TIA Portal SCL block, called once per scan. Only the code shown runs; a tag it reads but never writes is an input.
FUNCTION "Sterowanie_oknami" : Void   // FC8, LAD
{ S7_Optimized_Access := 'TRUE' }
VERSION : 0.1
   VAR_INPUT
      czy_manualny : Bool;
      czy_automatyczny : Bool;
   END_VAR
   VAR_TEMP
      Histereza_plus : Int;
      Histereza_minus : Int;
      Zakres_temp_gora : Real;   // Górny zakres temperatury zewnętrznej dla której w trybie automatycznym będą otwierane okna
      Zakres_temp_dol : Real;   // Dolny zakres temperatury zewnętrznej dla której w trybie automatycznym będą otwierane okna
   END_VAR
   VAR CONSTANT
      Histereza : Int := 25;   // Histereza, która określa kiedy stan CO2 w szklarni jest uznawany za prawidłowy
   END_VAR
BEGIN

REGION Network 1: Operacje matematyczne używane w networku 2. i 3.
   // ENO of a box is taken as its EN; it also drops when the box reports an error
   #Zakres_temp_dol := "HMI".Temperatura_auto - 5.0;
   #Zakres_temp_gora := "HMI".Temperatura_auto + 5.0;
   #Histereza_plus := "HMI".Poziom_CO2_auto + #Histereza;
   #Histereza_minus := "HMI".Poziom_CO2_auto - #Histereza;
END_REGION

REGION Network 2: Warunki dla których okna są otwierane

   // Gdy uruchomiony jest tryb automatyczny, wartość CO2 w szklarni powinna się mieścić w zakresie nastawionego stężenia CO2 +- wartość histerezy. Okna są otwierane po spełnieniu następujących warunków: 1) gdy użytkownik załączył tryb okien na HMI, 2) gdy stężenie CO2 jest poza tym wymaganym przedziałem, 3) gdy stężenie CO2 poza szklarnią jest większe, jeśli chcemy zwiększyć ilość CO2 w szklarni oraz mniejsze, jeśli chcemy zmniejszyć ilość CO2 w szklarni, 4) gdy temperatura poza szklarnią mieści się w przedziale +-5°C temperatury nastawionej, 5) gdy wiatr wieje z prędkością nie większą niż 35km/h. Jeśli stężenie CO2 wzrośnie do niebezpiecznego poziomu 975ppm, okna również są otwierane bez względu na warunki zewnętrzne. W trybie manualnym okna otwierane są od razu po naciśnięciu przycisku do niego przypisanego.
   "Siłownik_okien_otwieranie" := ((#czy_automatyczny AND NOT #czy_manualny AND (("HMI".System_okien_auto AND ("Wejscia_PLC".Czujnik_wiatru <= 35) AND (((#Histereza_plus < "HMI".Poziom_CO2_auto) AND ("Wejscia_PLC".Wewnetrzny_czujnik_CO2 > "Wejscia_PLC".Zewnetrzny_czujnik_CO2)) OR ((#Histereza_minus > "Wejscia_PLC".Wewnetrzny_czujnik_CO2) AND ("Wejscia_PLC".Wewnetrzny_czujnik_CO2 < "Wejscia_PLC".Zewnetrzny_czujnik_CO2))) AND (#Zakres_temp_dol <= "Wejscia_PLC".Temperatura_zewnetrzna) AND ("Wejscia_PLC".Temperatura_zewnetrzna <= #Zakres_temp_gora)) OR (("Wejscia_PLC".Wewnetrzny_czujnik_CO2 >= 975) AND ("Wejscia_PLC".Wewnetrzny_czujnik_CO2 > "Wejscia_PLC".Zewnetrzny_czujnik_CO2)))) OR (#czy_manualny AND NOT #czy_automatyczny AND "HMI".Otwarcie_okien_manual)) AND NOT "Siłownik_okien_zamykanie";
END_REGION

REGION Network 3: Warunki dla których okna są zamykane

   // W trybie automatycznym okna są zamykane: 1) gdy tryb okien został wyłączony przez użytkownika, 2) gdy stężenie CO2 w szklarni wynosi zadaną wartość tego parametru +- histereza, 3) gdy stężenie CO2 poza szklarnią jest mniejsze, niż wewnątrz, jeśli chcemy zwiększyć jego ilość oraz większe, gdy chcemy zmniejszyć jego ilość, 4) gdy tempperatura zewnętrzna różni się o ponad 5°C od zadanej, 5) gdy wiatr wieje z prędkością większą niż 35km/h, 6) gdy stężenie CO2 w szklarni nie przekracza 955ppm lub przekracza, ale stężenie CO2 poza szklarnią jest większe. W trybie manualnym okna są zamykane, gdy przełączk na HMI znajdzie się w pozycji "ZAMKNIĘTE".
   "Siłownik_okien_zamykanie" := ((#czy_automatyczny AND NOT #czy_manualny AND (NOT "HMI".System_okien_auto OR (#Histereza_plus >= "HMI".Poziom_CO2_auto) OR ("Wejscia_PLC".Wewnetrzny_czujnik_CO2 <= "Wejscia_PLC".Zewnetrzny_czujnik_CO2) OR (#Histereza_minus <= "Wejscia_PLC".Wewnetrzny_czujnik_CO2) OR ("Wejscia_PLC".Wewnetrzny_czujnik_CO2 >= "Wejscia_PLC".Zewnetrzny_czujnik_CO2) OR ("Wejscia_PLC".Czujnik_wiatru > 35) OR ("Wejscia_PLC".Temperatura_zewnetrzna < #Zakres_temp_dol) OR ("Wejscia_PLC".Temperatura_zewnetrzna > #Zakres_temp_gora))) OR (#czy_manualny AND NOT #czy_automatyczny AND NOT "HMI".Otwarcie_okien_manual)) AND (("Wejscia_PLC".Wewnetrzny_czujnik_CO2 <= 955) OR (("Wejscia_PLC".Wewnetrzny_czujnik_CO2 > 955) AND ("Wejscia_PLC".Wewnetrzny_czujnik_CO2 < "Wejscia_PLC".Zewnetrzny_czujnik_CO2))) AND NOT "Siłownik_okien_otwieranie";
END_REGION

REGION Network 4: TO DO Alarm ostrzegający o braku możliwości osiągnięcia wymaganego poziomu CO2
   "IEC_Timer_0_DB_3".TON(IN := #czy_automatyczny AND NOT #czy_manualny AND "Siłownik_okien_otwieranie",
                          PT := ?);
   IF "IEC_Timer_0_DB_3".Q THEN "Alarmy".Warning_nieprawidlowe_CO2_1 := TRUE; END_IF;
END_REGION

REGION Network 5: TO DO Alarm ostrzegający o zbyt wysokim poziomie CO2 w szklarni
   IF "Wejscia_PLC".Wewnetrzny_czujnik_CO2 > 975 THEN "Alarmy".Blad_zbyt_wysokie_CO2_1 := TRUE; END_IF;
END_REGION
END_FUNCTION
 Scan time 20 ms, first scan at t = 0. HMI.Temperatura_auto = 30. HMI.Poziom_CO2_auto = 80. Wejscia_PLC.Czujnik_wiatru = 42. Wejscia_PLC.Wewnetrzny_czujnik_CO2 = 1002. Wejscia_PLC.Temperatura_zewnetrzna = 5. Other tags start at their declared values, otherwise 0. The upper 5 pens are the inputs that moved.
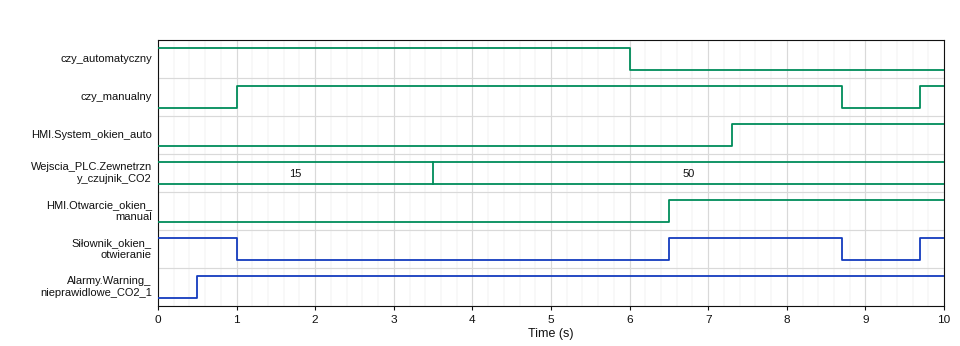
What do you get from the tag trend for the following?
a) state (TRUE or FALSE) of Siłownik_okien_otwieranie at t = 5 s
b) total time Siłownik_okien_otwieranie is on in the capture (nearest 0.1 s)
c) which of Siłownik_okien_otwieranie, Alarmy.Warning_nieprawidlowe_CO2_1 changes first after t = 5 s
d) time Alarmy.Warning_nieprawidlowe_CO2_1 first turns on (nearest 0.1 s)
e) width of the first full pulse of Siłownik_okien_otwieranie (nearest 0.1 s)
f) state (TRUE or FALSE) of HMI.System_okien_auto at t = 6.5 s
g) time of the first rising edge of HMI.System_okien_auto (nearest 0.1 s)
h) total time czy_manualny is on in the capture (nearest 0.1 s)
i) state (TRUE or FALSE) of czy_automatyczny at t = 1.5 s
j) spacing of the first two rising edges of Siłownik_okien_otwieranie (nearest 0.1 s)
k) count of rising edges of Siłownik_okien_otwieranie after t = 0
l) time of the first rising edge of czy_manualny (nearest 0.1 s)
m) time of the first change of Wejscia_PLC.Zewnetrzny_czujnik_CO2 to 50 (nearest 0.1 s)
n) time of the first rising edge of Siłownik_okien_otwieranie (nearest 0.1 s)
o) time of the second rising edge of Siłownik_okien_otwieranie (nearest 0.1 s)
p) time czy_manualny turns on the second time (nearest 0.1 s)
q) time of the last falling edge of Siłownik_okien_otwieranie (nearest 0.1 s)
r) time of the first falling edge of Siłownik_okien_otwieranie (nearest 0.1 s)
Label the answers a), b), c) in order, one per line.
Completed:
a) FALSE
b) 3.5 s
c) Siłownik_okien_otwieranie
d) 0.5 s
e) 2.2 s
f) FALSE
g) 7.3 s
h) 8.0 s
i) TRUE
j) 3.2 s
k) 2
l) 1.0 s
m) 3.5 s
n) 6.5 s
o) 9.7 s
p) 9.7 s
q) 8.7 s
r) 1.0 s
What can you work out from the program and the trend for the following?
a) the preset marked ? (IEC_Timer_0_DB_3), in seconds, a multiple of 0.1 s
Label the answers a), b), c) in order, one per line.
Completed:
a) 0.5 s
